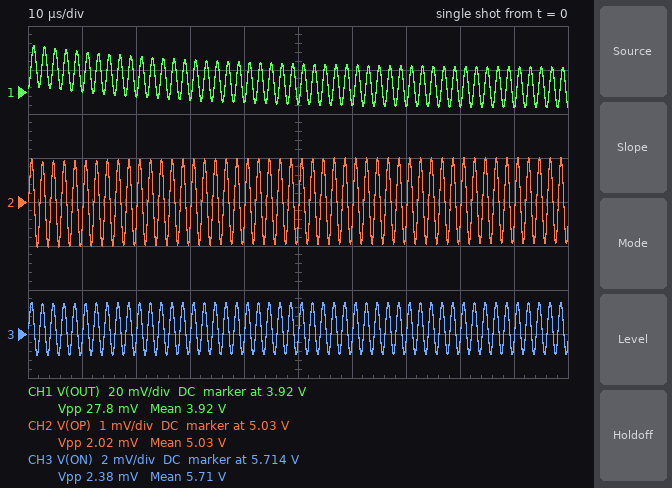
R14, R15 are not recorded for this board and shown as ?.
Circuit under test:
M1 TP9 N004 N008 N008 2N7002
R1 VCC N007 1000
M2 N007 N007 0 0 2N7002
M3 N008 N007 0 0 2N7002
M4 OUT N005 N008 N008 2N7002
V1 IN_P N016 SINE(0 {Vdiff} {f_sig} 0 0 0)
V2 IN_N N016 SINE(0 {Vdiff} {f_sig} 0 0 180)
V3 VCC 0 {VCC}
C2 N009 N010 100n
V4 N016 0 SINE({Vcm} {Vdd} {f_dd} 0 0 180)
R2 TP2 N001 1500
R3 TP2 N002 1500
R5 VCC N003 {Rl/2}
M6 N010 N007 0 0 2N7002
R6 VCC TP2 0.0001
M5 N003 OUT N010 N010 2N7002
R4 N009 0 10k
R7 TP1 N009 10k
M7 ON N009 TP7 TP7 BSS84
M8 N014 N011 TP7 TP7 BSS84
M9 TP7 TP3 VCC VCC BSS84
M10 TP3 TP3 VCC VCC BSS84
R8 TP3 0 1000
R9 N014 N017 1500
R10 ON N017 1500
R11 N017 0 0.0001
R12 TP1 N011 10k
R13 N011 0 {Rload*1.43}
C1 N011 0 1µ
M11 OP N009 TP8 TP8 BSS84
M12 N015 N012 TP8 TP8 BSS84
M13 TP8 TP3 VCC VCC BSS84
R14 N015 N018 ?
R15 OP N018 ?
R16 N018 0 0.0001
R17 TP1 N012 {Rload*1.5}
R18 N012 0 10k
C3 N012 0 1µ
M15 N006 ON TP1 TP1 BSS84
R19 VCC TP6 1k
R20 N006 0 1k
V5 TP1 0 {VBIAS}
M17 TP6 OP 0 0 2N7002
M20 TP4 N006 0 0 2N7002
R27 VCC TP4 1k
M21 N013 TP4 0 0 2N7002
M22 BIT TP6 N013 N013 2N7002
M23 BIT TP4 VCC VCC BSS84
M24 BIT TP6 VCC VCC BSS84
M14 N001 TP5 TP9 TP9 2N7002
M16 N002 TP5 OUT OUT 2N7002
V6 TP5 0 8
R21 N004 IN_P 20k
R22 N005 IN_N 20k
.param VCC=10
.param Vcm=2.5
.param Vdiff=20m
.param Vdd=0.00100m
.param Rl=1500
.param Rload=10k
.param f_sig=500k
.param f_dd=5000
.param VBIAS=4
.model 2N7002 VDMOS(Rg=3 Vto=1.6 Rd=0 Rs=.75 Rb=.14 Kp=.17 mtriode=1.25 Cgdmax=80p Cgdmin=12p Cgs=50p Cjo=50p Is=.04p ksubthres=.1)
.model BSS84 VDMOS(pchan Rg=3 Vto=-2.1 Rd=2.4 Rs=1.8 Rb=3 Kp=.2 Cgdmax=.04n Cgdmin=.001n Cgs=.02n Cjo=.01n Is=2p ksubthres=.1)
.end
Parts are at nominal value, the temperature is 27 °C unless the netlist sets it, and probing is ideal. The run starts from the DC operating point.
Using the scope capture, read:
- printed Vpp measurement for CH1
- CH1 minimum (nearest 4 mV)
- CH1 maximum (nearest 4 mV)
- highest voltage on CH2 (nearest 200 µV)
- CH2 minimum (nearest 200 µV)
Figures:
27.8 mV
3.912 V
3.940 V
5.0310 V
5.0290 V
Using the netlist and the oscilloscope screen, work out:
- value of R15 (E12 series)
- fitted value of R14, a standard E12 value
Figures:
3.3 kΩ
820 Ω
